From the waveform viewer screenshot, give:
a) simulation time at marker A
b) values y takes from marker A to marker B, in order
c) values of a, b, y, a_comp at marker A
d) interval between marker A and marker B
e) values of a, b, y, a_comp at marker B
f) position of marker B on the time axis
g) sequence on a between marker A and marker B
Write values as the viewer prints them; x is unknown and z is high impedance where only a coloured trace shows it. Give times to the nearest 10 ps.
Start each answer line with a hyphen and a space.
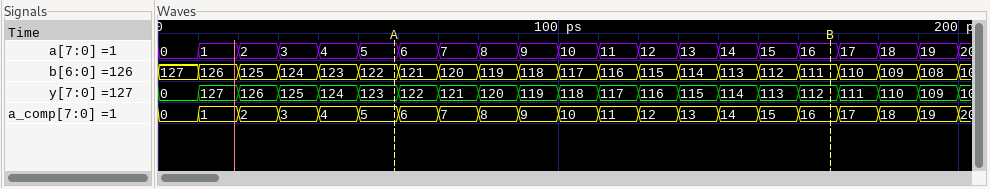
- 60 ps
- 123, 122, 121, 120, 119, 118, 117, 116, 115, 114, 113, 112
- a=5, b=122, y=123, a_comp=5
- 110 ps
- a=16, b=111, y=112, a_comp=16
- 170 ps
- 5, 6, 7, 8, 9, 10, 11, 12, 13, 14, 15, 16
